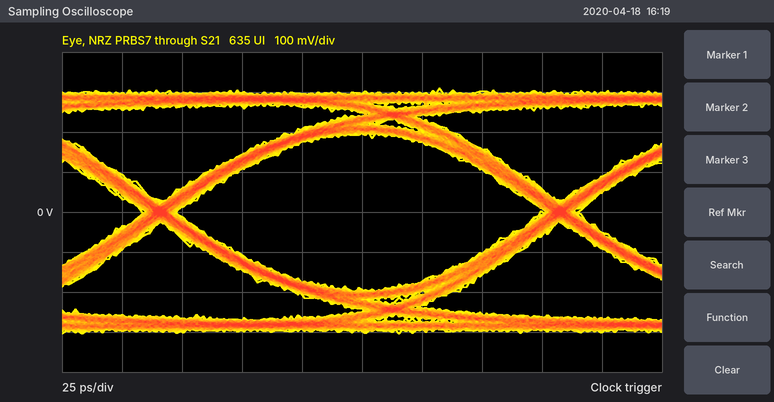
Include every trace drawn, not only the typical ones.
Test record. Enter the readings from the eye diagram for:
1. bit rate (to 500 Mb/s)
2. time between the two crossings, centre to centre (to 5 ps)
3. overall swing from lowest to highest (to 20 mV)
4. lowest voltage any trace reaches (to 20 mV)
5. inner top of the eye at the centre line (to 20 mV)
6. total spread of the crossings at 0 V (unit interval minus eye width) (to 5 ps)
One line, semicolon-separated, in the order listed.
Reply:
6.0 Gb/s; 165 ps; 620 mV; -300 mV; 200 mV; 15 ps
